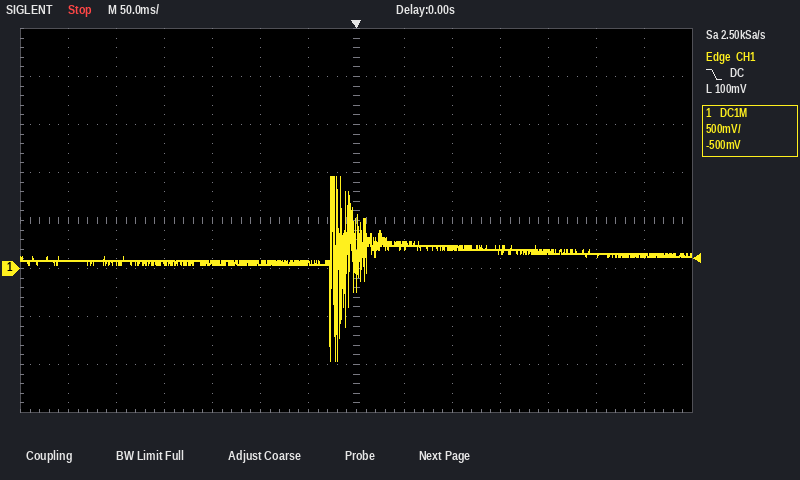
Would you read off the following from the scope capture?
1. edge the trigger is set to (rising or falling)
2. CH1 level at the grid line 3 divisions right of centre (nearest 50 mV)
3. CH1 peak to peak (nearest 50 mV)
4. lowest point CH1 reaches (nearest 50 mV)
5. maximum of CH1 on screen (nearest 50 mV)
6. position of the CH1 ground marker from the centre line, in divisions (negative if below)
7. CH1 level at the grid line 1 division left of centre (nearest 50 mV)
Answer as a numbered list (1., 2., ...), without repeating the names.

1. falling
2. 200 mV
3. 1.90 V
4. -950 mV
5. 950 mV
6. -1.0 div
7. 50 mV
